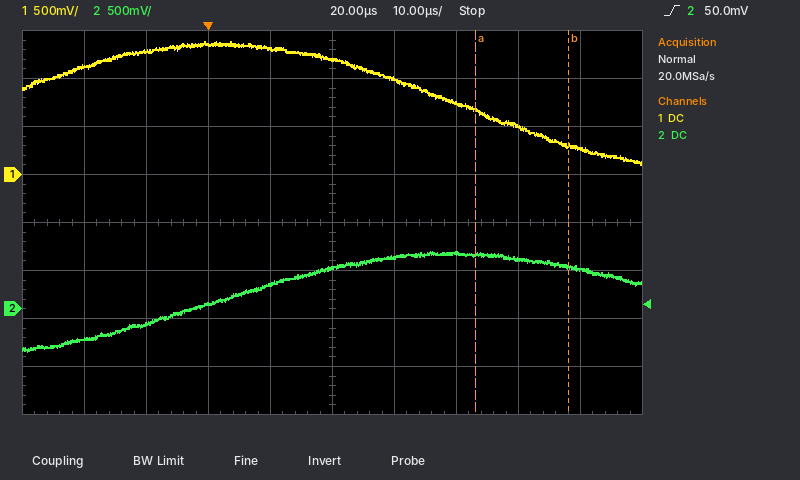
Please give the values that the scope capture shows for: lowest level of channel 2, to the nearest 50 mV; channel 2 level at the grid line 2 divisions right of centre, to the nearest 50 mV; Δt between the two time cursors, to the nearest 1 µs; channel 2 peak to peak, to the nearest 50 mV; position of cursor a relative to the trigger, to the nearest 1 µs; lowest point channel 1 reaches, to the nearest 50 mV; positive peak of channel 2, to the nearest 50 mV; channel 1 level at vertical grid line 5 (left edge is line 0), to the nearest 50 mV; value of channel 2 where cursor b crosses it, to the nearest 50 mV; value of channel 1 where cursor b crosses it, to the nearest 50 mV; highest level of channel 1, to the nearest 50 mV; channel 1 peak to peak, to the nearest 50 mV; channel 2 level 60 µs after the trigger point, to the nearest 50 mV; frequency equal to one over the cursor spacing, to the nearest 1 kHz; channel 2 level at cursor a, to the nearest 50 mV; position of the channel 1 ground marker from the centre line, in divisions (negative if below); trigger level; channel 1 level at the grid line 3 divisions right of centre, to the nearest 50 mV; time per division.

-450 mV
600 mV
15 µs
1.05 V
+43 µs
100 mV
600 mV
1.20 V
450 mV
300 mV
1.40 V
1.30 V
400 mV
67 kHz
550 mV
+1.0 div
50.0 mV
500 mV
10 µs
